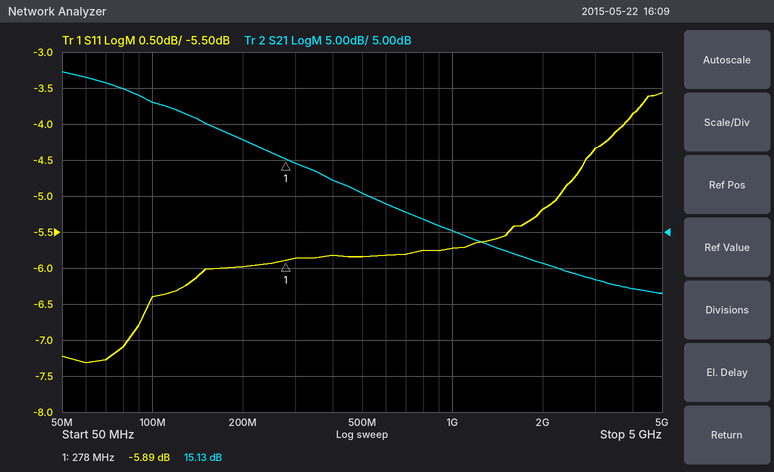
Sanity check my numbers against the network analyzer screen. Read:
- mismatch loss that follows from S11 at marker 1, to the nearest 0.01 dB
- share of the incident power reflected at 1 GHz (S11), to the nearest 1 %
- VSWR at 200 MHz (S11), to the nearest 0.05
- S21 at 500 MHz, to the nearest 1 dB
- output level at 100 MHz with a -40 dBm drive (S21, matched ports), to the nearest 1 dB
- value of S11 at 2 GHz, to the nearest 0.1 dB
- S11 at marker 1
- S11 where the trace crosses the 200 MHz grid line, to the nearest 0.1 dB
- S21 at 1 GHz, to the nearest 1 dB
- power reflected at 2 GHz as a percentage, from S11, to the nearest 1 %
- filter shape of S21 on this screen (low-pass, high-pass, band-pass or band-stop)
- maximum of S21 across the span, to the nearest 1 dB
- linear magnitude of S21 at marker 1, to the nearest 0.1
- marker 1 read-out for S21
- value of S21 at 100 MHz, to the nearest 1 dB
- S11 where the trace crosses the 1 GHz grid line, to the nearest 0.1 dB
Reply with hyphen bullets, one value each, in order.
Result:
- 1.29 dB
- 27 %
- 3.00
- 10 dB
- -17 dBm
- -5.2 dB
- -5.89 dB
- -6.0 dB
- 5 dB
- 30 %
- low-pass
- 27 dB
- 5.7
- 15.13 dB
- 23 dB
- -5.7 dB
